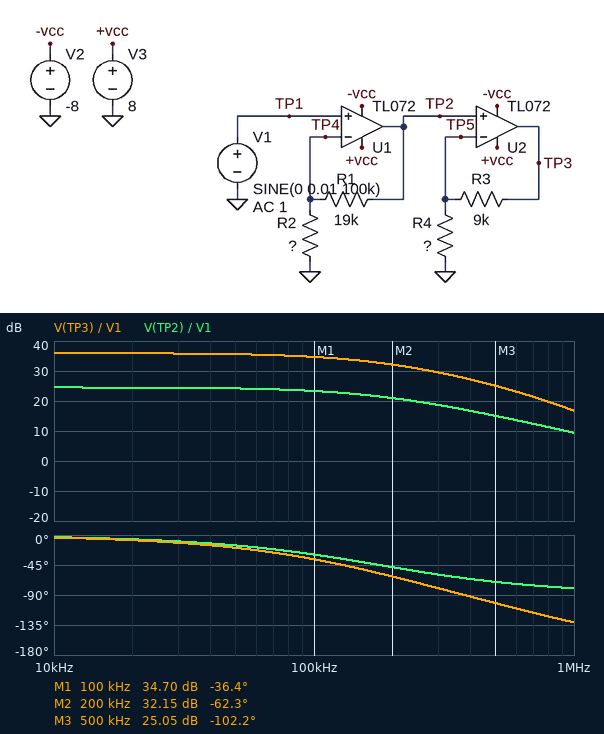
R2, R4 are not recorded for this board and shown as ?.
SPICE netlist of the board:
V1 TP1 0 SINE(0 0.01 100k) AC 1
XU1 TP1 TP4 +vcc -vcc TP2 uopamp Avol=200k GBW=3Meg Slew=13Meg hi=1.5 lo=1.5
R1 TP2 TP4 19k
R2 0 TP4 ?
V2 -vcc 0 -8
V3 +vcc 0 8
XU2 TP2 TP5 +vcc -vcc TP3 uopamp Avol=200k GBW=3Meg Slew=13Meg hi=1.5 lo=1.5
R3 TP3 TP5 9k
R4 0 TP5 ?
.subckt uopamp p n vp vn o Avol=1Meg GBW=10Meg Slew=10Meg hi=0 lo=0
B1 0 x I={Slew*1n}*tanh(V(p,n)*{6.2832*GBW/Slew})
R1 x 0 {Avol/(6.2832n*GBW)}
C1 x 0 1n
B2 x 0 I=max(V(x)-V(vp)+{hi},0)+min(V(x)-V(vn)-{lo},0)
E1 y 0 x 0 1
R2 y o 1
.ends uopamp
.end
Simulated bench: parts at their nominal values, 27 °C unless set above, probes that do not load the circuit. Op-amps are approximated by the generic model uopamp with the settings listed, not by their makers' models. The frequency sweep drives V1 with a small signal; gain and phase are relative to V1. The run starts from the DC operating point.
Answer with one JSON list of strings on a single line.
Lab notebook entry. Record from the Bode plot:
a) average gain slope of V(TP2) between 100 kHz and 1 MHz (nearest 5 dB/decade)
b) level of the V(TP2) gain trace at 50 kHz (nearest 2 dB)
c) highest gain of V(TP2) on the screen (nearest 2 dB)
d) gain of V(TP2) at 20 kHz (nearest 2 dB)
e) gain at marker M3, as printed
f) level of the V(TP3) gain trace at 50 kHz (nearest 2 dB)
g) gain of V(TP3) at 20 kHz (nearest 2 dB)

["-15 dB/decade", "24 dB", "24 dB", "24 dB", "25.05 dB", "36 dB", "36 dB"]
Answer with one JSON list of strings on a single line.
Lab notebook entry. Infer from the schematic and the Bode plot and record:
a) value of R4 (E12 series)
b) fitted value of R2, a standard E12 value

["3.3 kΩ", "1.2 kΩ"]
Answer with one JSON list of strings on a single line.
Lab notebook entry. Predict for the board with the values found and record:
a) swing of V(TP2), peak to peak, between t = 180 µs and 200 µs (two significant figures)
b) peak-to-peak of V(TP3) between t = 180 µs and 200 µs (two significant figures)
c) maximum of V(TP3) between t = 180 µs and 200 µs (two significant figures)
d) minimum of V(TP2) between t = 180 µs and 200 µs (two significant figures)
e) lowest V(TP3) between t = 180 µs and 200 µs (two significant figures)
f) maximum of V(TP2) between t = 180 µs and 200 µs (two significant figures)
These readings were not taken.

["290 mV", "1.1 V", "540 mV", "-150 mV", "-540 mV", "150 mV"]
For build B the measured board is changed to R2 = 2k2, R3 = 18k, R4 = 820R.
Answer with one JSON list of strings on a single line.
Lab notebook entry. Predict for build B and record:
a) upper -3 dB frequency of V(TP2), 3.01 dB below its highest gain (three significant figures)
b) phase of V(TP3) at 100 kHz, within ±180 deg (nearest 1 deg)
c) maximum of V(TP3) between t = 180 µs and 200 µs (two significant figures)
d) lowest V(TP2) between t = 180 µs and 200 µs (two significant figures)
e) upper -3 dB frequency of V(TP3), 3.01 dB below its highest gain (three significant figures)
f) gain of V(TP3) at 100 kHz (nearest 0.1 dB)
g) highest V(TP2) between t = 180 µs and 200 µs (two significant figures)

["311 kHz", "-55 deg", "1.7 V", "-92 mV", "114 kHz", "44.5 dB", "92 mV"]
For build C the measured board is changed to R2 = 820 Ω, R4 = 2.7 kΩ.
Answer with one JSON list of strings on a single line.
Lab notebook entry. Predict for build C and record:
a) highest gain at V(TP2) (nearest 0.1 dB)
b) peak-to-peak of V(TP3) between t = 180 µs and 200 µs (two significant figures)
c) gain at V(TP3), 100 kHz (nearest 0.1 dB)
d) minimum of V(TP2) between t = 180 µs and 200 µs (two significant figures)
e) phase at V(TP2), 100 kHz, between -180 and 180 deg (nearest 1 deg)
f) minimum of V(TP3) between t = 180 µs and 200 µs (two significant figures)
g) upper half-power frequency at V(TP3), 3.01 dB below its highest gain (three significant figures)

["27.7 dB", "1.6 V", "38.1 dB", "-190 mV", "-39 deg", "-810 mV", "120 kHz"]
